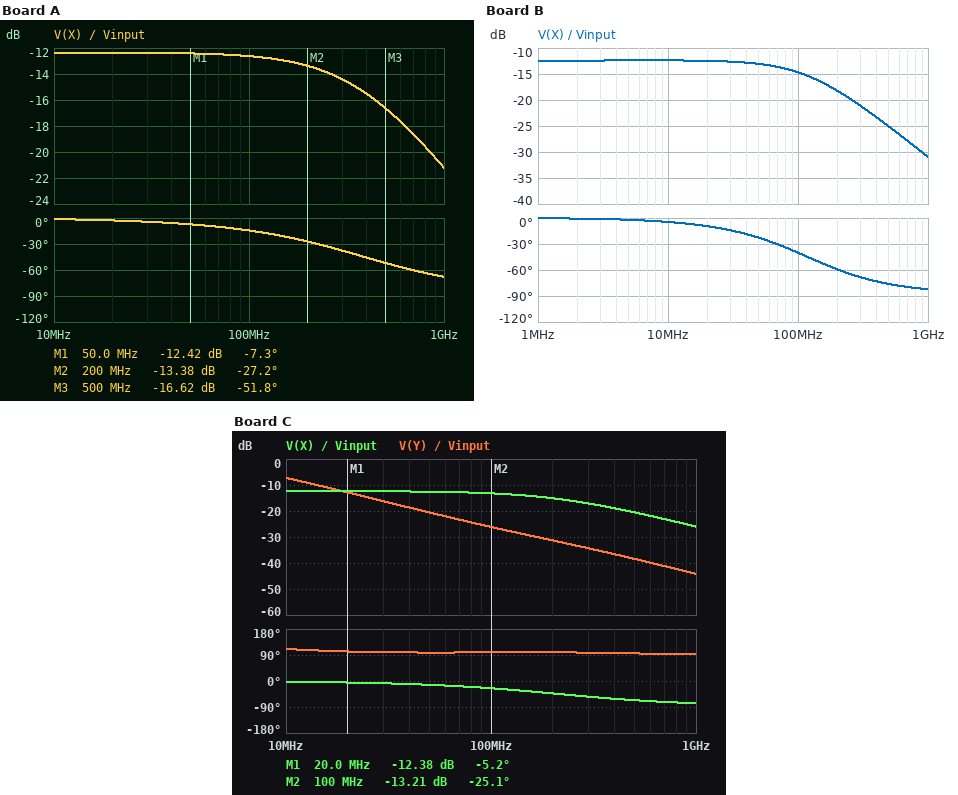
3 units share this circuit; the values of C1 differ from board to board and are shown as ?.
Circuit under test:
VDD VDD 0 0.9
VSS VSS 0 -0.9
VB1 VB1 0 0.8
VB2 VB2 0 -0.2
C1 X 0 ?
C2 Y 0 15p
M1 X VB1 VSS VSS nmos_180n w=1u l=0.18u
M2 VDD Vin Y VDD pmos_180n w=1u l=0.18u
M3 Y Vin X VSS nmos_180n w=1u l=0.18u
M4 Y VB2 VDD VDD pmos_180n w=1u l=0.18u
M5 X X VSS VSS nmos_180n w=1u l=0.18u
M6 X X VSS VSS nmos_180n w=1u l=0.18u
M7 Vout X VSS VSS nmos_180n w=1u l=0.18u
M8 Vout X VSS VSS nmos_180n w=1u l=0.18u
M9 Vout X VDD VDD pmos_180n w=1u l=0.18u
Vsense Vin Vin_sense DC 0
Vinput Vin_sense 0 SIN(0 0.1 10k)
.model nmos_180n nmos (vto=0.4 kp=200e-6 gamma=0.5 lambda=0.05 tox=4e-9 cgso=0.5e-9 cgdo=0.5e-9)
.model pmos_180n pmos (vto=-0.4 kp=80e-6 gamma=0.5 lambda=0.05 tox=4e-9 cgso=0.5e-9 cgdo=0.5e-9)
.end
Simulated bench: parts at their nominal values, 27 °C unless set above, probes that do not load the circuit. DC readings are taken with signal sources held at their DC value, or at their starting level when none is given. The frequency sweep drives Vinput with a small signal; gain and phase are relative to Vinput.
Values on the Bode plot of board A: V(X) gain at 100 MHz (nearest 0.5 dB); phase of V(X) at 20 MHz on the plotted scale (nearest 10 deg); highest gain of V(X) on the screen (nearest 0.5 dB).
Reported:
-12.5 dB
0 deg
-12.5 dB
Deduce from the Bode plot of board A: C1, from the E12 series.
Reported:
820 fF
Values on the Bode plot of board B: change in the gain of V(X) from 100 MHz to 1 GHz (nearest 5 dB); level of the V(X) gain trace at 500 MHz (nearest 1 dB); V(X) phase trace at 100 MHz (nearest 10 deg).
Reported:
-15 dB
-25 dB
-40 deg
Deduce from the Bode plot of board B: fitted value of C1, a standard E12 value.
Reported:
2.7 pF
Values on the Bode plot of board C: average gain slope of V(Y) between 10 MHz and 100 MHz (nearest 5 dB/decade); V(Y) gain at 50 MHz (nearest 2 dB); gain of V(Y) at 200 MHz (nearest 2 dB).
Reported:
-20 dB/decade
-20 dB
-32 dB
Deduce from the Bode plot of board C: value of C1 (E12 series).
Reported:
1.5 pF
